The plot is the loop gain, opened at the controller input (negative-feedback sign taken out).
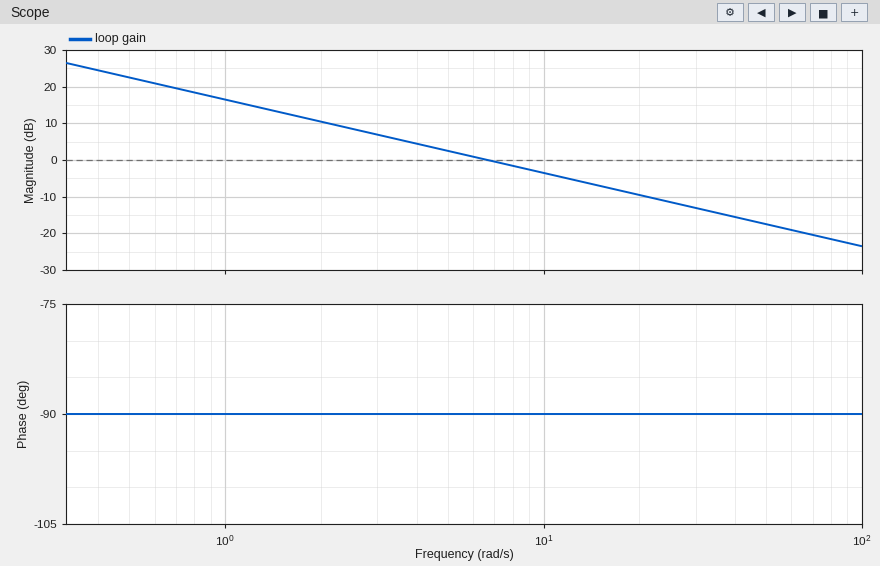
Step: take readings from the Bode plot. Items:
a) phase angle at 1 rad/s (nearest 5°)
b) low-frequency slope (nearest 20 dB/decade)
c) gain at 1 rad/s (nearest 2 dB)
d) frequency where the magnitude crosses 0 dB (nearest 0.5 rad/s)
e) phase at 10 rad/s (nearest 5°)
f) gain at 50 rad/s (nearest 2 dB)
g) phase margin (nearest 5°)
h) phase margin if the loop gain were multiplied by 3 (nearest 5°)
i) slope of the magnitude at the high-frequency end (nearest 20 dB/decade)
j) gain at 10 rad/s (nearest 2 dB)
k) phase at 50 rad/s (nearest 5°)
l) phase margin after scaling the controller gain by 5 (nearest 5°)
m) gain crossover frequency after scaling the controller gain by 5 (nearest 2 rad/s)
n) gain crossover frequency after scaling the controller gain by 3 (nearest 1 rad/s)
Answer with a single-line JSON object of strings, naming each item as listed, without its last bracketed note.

{"phase angle at 1 rad/s": "-90°", "low-frequency slope": "-20 dB/decade", "gain at 1 rad/s": "16 dB", "frequency where the magnitude crosses 0 dB": "6.5 rad/s", "phase at 10 rad/s": "-90°", "gain at 50 rad/s": "-18 dB", "phase margin": "90°", "phase margin if the loop gain were multiplied by 3": "90°", "slope of the magnitude at the high-frequency end": "-20 dB/decade", "gain at 10 rad/s": "-4 dB", "phase at 50 rad/s": "-90°", "phase margin after scaling the controller gain by 5": "90°", "gain crossover frequency after scaling the controller gain by 5": "34 rad/s", "gain crossover frequency after scaling the controller gain by 3": "20 rad/s"}
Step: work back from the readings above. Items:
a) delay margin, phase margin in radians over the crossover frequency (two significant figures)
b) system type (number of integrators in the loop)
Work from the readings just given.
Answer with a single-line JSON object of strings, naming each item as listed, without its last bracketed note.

{"delay margin, phase margin in radians over the crossover frequency": "0.24 s", "system type": "1"}
